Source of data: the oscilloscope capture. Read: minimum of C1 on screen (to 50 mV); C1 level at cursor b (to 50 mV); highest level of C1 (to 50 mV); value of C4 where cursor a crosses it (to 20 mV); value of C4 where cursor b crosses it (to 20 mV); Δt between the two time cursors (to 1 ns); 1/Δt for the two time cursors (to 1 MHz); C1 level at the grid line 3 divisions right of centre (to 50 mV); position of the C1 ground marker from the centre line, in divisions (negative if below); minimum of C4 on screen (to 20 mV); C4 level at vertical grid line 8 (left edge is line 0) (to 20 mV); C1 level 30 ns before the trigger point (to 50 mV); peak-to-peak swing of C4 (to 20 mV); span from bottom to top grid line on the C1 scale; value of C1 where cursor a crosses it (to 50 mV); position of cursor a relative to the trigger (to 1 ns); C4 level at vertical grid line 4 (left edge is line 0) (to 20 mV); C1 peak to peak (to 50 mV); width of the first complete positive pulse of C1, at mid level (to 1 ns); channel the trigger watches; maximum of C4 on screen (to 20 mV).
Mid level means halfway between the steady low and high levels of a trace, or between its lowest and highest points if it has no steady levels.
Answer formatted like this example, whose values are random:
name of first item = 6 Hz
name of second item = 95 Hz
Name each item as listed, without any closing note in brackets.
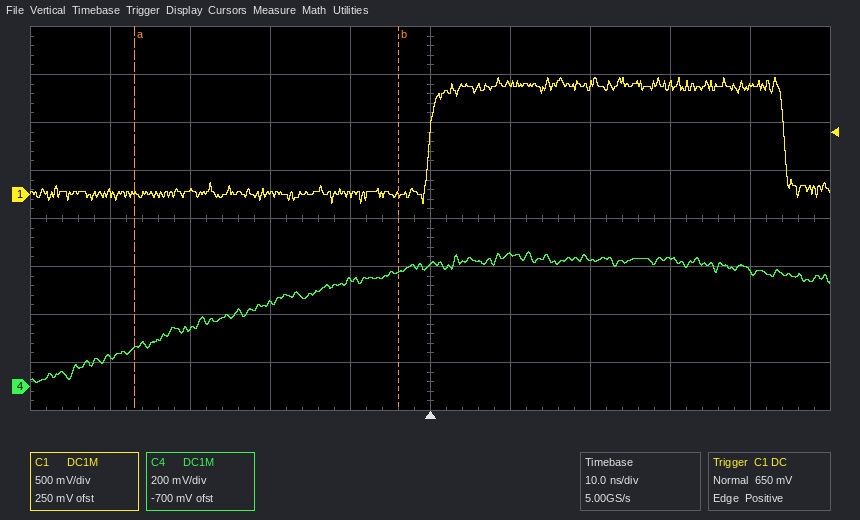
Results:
minimum of C1 on screen = -100 mV
C1 level at cursor b = 0 mV
highest level of C1 = 1.20 V
value of C4 where cursor a crosses it = 160 mV
value of C4 where cursor b crosses it = 480 mV
Δt between the two time cursors = 33 ns
1/Δt for the two time cursors = 30 MHz
C1 level at the grid line 3 divisions right of centre = 1.15 V
position of the C1 ground marker from the centre line, in divisions = +0.5 div
minimum of C4 on screen = 20 mV
C4 level at vertical grid line 8 (left edge is line 0) = 540 mV
C1 level 30 ns before the trigger point = 50 mV
peak-to-peak swing of C4 = 540 mV
span from bottom to top grid line on the C1 scale = 4 V
value of C1 where cursor a crosses it = 0 mV
position of cursor a relative to the trigger = -37 ns
C4 level at vertical grid line 4 (left edge is line 0) = 440 mV
C1 peak to peak = 1.30 V
width of the first complete positive pulse of C1, at mid level = 44 ns
channel the trigger watches = C1
maximum of C4 on screen = 560 mV
